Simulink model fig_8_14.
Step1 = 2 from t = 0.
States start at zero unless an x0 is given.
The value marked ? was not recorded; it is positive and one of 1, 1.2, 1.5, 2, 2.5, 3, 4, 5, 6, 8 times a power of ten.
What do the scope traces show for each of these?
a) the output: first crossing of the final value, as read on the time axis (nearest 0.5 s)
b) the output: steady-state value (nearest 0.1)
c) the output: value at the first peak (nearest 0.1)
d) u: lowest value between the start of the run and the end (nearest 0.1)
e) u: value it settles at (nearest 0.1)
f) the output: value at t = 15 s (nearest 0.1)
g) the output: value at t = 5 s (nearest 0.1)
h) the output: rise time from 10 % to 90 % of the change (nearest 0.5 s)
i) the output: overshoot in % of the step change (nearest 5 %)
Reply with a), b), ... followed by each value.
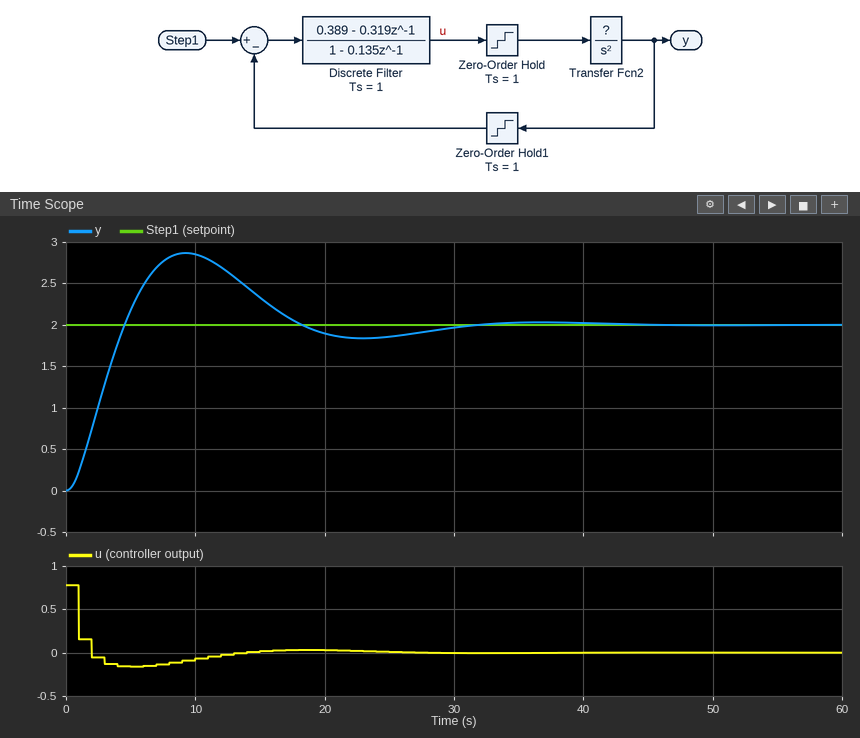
a) 4.5 s
b) 2.0
c) 2.9
d) -0.2
e) 0.0
f) 2.3
g) 2.2
h) 3.0 s
i) 45 %
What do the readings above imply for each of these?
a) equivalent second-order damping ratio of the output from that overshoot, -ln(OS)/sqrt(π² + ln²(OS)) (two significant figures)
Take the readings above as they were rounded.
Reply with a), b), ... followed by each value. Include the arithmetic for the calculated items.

a) ln(0.45) = -0.799; 0.799 / sqrt(9.870 + 0.638) = 0.25
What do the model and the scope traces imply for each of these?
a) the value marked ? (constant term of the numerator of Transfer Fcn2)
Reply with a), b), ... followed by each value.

a) 0.6
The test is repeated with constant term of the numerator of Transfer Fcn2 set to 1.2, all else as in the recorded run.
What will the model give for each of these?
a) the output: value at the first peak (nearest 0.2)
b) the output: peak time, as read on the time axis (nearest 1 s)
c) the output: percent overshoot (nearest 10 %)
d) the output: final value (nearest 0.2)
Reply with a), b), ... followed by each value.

a) 3.0
b) 5 s
c) 50 %
d) 2.0
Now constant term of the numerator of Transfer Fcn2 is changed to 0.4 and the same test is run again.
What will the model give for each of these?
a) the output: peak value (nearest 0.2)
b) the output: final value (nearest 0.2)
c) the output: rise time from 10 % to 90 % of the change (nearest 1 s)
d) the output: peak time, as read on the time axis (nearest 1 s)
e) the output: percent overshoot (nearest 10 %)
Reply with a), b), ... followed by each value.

a) 3.0
b) 2.0
c) 4 s
d) 13 s
e) 50 %
